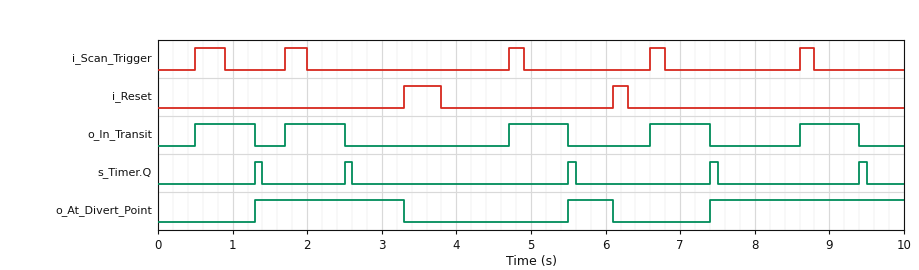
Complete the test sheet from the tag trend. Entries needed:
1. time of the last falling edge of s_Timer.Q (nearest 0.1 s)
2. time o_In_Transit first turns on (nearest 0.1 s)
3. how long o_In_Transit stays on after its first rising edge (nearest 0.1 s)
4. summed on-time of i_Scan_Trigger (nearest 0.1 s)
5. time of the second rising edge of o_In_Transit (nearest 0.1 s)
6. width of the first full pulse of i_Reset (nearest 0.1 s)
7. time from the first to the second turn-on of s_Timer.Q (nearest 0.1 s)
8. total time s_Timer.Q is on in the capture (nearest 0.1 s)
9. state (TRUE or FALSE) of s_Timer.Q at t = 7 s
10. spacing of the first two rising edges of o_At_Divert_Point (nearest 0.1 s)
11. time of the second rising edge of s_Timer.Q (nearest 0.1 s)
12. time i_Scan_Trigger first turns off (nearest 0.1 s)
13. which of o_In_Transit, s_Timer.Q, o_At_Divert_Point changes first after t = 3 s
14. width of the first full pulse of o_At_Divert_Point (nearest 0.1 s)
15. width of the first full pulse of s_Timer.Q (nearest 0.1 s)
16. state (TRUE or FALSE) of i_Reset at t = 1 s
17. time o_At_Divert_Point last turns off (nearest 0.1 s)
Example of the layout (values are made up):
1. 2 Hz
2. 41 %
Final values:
1. 9.5 s
2. 0.5 s
3. 0.8 s
4. 1.3 s
5. 1.7 s
6. 0.5 s
7. 1.2 s
8. 0.5 s
9. FALSE
10. 4.2 s
11. 2.5 s
12. 0.9 s
13. o_At_Divert_Point
14. 2.0 s
15. 0.1 s
16. FALSE
17. 6.1 s
